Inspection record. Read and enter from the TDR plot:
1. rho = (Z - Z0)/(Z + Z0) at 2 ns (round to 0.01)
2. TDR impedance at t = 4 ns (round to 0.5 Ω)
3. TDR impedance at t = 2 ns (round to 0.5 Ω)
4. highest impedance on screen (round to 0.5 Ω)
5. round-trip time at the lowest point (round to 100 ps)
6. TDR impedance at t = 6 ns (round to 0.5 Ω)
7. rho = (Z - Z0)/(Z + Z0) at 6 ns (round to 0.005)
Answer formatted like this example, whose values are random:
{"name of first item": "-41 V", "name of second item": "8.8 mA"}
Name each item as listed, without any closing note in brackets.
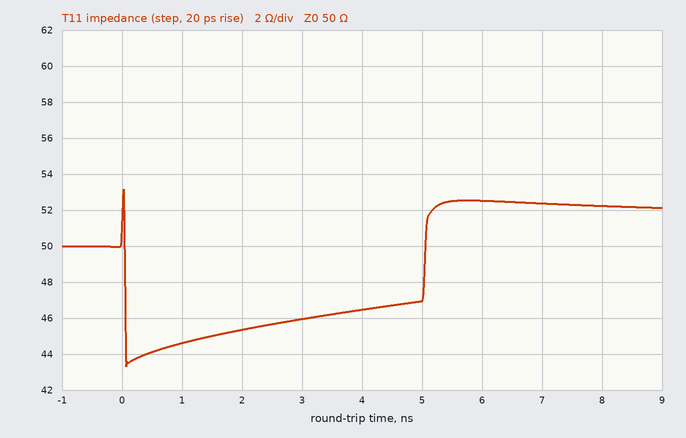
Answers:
{"rho = (Z - Z0)/(Z + Z0) at 2 ns": "-0.05", "TDR impedance at t = 4 ns": "46.5 Ω", "TDR impedance at t = 2 ns": "45.5 Ω", "highest impedance on screen": "53.0 Ω", "round-trip time at the lowest point": "100 ps", "TDR impedance at t = 6 ns": "52.5 Ω", "rho = (Z - Z0)/(Z + Z0) at 6 ns": "+0.025"}
